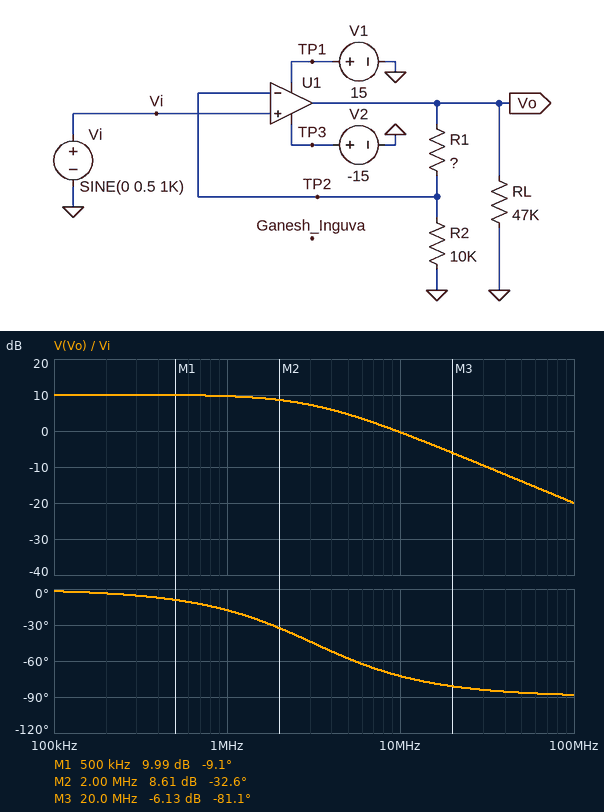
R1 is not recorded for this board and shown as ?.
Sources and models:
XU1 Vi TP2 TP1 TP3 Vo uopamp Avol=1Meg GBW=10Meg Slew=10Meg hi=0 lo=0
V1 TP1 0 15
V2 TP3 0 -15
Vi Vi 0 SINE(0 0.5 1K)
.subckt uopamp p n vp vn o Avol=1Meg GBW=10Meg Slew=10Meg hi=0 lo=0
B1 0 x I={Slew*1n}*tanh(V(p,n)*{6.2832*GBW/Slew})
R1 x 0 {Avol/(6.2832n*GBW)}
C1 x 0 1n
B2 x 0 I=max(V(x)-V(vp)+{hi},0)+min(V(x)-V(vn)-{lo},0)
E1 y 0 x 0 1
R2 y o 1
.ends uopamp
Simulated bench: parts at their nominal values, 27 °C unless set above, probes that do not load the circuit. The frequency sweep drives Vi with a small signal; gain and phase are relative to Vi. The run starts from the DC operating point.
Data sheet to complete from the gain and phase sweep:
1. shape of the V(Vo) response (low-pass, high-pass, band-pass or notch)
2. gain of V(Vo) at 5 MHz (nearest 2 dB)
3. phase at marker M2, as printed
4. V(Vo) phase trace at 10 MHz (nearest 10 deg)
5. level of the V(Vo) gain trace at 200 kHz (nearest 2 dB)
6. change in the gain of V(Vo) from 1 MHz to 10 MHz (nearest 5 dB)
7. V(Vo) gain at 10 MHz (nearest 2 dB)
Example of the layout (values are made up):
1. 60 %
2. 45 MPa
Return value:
1. low-pass
2. 4 dB
3. -32.6 deg
4. -70 deg
5. 10 dB
6. -10 dB
7. 0 dB
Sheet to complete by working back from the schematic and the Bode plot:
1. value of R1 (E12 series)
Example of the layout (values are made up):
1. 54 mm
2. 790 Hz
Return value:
1. 22 kΩ
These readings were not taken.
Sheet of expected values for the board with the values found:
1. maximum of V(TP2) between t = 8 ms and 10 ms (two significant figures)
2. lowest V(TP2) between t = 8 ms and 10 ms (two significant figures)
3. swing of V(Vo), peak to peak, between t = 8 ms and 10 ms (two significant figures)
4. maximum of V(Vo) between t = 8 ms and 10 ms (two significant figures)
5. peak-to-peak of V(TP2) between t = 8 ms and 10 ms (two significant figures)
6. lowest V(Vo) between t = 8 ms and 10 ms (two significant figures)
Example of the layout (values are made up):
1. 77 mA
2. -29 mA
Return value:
1. 500 mV
2. -500 mV
3. 3.2 V
4. 1.6 V
5. 1.0 V
6. -1.6 V
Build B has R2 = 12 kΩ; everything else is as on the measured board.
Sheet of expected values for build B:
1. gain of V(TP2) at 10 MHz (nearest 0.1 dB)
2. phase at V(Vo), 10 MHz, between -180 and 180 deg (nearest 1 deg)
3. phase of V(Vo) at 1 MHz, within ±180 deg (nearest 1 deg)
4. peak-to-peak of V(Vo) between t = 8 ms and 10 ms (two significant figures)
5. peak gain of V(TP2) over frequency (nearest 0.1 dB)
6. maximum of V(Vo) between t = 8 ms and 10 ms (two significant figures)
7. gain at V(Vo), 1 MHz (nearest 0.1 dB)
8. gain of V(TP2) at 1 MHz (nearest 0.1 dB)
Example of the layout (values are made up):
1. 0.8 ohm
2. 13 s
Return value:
1. -9.6 dB
2. -71 deg
3. -16 deg
4. 2.8 V
5. 0 dB
6. 1.4 V
7. 8.7 dB
8. -0.3 dB
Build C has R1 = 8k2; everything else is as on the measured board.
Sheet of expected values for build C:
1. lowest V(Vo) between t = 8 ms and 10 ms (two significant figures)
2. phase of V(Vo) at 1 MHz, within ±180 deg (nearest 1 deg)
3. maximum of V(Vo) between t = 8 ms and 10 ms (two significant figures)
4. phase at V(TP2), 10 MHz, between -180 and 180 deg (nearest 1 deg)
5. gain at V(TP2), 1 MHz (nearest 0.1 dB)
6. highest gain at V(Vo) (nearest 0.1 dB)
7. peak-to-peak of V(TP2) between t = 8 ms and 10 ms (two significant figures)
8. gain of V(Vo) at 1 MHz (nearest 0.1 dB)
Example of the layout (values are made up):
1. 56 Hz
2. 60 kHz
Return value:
1. -910 mV
2. -10 deg
3. 910 mV
4. -61 deg
5. -0.1 dB
6. 5.2 dB
7. 1.0 V
8. 5.1 dB
